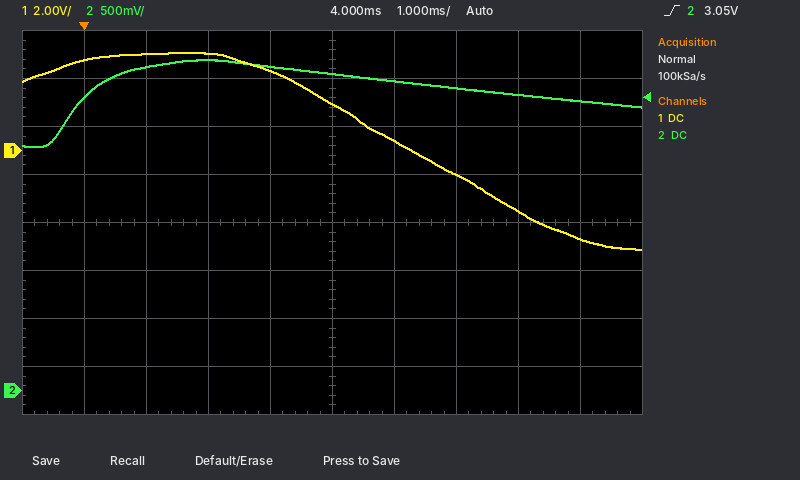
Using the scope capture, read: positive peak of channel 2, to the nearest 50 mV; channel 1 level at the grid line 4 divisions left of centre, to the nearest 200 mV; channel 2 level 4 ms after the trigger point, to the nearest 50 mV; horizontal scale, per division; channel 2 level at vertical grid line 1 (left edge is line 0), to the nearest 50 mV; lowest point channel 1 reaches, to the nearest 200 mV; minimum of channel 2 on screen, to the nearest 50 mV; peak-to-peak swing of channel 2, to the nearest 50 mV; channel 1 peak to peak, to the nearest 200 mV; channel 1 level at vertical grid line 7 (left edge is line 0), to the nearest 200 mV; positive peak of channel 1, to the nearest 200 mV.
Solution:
3.45 V
3.8 V
3.30 V
1 ms
3.05 V
-4.2 V
2.55 V
900 mV
8.2 V
-1.0 V
4.0 V
